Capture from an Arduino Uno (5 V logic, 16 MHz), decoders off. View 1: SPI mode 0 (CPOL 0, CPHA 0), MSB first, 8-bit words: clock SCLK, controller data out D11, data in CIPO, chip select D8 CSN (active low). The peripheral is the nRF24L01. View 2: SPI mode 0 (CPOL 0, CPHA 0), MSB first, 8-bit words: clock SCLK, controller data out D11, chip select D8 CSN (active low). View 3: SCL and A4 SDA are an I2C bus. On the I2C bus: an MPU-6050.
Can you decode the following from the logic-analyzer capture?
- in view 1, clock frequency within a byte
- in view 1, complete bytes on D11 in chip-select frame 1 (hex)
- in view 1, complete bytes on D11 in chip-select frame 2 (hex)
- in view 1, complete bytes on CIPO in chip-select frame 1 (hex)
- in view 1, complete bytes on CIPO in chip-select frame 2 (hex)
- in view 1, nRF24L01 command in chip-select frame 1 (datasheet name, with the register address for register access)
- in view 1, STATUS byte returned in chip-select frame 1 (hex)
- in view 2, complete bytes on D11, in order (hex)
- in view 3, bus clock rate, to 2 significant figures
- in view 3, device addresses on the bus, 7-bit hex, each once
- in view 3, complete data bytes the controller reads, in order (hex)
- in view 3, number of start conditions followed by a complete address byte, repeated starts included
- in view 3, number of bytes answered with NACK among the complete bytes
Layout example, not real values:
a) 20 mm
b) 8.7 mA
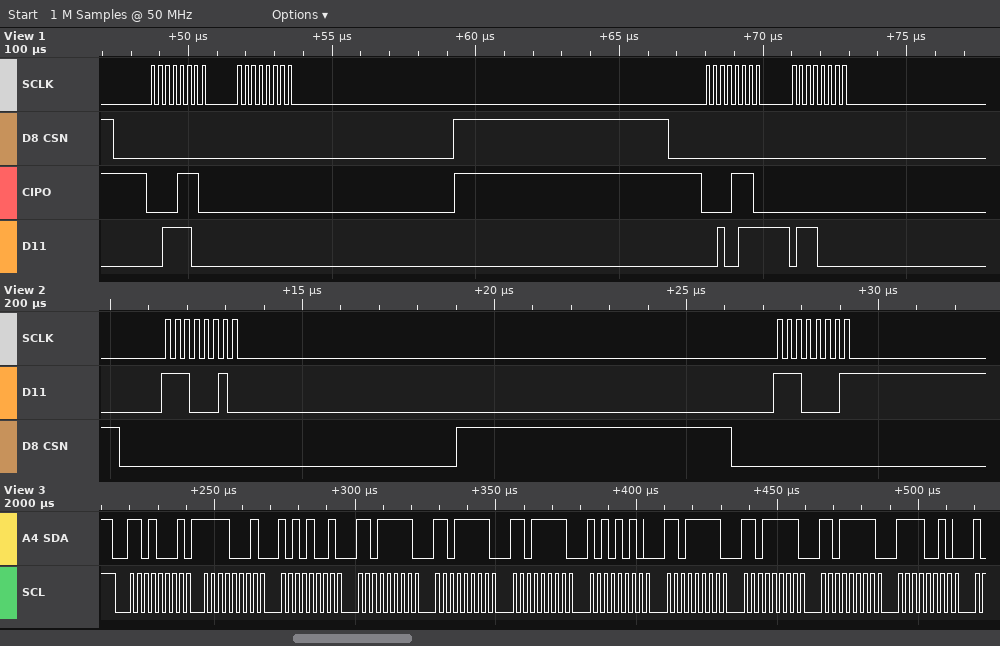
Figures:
a) 4 MHz
b) 0x3C 0x00
c) 0x27 0x70
d) 0x0E 0x00
e) 0x0E 0x00
f) W_REGISTER 0x1C
g) 0x0E
h) E2 E1
i) 400 kHz
j) 0x68
k) F1 A9 DF DF DF AA DF DF DF F2
l) 1
m) 0
